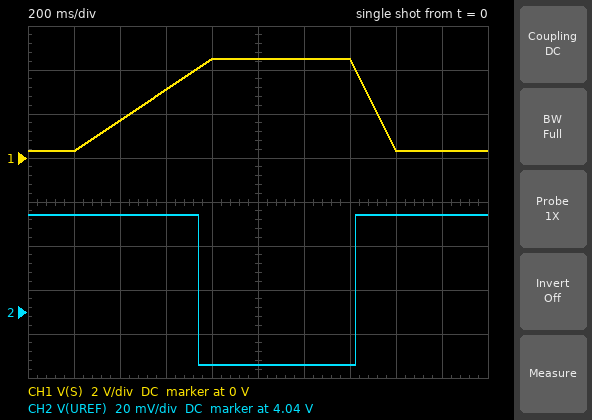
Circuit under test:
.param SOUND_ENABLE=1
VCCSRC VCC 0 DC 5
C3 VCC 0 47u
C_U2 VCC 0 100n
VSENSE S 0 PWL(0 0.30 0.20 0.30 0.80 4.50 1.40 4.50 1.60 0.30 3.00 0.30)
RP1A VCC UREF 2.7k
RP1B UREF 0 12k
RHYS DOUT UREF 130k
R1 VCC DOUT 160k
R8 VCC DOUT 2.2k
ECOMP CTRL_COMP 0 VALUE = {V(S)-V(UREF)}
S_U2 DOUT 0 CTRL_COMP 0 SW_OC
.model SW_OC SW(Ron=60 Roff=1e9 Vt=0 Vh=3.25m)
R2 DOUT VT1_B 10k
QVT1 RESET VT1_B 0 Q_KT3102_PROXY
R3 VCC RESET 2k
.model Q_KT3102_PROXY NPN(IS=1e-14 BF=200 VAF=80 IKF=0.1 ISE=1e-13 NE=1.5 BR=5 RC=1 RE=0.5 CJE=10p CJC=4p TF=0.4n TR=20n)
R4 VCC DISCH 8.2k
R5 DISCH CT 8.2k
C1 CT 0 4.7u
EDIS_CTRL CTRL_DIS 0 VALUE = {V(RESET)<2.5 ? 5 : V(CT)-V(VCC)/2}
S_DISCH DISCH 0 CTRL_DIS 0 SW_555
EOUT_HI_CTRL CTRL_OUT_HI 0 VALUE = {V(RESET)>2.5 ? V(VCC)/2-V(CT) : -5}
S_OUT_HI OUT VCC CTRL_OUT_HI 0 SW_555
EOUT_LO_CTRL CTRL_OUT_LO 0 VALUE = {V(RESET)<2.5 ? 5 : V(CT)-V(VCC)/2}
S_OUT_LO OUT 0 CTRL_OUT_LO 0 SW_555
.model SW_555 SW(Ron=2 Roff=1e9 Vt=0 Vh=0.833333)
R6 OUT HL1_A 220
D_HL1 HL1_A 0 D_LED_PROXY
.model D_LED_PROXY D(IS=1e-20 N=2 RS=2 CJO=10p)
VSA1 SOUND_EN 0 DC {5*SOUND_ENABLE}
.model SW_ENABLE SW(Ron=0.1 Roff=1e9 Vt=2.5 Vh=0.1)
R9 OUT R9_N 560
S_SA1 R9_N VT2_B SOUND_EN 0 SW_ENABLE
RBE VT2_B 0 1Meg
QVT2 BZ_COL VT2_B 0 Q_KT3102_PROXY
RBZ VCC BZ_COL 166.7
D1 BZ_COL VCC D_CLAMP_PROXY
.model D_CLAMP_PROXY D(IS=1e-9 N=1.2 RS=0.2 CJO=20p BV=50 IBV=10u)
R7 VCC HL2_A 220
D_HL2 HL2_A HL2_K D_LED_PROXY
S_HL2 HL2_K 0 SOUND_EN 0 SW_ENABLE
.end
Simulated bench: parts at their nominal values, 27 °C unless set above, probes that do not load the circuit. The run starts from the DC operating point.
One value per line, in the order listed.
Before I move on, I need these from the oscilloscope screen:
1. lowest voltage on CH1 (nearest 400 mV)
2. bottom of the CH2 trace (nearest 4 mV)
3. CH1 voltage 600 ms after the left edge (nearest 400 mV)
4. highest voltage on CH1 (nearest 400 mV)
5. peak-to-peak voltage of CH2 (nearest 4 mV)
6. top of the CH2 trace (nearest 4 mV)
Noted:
400 mV
4.016 V
3.2 V
4.4 V
68 mV
4.084 V
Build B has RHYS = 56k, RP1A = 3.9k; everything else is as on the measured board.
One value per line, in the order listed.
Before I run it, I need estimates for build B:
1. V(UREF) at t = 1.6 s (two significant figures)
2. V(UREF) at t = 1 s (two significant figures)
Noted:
3.8 V
3.6 V
